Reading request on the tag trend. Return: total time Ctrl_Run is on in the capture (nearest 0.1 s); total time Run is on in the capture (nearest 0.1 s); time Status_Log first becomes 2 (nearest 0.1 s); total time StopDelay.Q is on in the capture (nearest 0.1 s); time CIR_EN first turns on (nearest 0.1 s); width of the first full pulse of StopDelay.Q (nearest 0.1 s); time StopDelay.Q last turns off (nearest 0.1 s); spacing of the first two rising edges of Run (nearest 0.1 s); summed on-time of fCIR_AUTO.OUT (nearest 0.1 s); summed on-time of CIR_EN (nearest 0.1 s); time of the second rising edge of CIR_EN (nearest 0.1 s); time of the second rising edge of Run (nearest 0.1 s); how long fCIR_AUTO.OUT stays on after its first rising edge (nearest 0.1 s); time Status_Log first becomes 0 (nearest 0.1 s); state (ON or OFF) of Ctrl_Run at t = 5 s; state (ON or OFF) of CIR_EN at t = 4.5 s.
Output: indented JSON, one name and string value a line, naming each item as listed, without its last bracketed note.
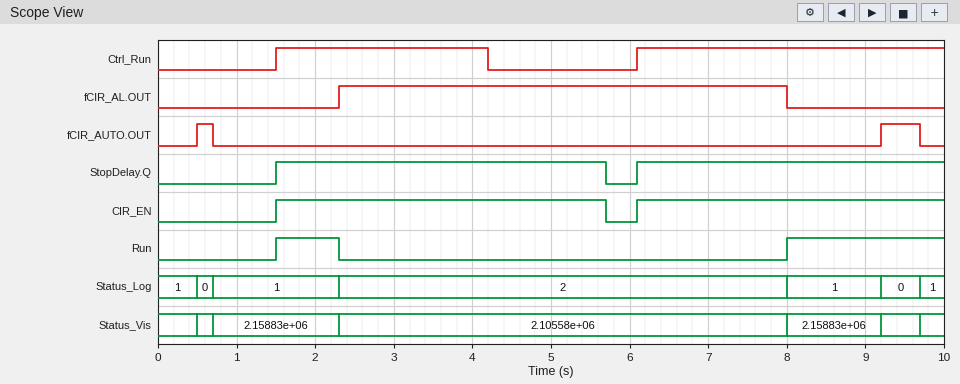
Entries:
{
  "total time Ctrl_Run is on in the capture": "6.6 s",
  "total time Run is on in the capture": "2.8 s",
  "time Status_Log first becomes 2": "2.3 s",
  "total time StopDelay.Q is on in the capture": "8.1 s",
  "time CIR_EN first turns on": "1.5 s",
  "width of the first full pulse of StopDelay.Q": "4.2 s",
  "time StopDelay.Q last turns off": "5.7 s",
  "spacing of the first two rising edges of Run": "6.5 s",
  "summed on-time of fCIR_AUTO.OUT": "0.7 s",
  "summed on-time of CIR_EN": "8.1 s",
  "time of the second rising edge of CIR_EN": "6.1 s",
  "time of the second rising edge of Run": "8.0 s",
  "how long fCIR_AUTO.OUT stays on after its first rising edge": "0.2 s",
  "time Status_Log first becomes 0": "0.5 s",
  "state (ON or OFF) of Ctrl_Run at t = 5 s": "OFF",
  "state (ON or OFF) of CIR_EN at t = 4.5 s": "ON"
}
